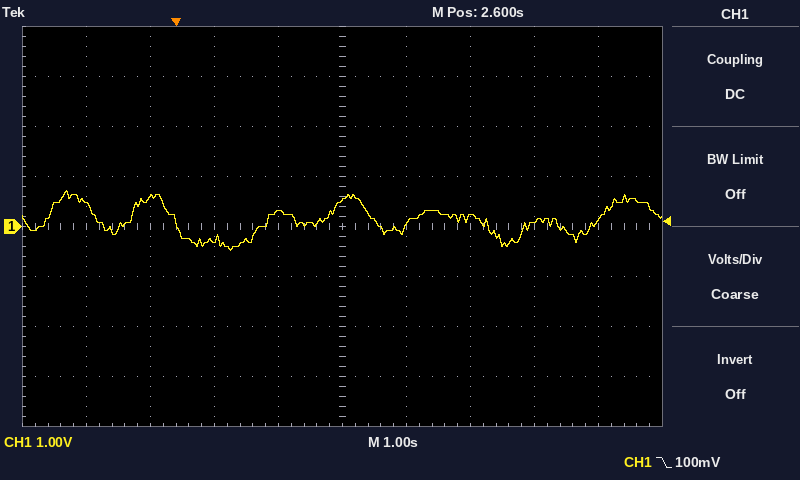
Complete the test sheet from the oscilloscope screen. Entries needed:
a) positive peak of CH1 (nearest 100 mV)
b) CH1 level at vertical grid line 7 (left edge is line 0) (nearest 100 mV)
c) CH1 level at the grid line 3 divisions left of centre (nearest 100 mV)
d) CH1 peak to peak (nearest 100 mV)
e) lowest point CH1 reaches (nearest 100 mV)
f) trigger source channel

700 mV
200 mV
600 mV
1.2 V
-500 mV
CH1
